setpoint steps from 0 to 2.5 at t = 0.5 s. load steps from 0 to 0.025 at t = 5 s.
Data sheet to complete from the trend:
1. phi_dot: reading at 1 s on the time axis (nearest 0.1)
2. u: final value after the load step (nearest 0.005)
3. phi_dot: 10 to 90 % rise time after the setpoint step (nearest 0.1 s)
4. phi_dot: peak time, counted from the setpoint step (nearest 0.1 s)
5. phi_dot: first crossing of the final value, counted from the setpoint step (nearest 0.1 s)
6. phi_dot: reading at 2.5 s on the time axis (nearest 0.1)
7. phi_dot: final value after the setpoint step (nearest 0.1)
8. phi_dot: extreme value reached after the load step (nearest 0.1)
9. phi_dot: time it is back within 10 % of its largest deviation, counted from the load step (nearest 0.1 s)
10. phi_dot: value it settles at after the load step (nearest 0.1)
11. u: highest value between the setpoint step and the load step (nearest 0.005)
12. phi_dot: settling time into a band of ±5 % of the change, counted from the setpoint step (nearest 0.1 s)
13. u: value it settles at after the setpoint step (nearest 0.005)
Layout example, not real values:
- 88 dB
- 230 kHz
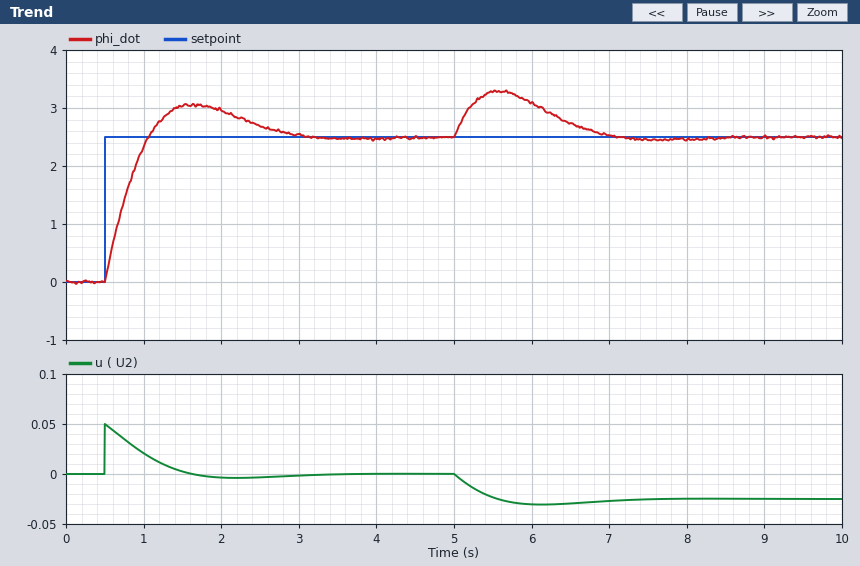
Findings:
- 2.3
- -0.025
- 0.4 s
- 1.1 s
- 0.6 s
- 2.7
- 2.5
- 3.3
- 1.8 s
- 2.5
- 0.050
- 2.2 s
- 0.000
